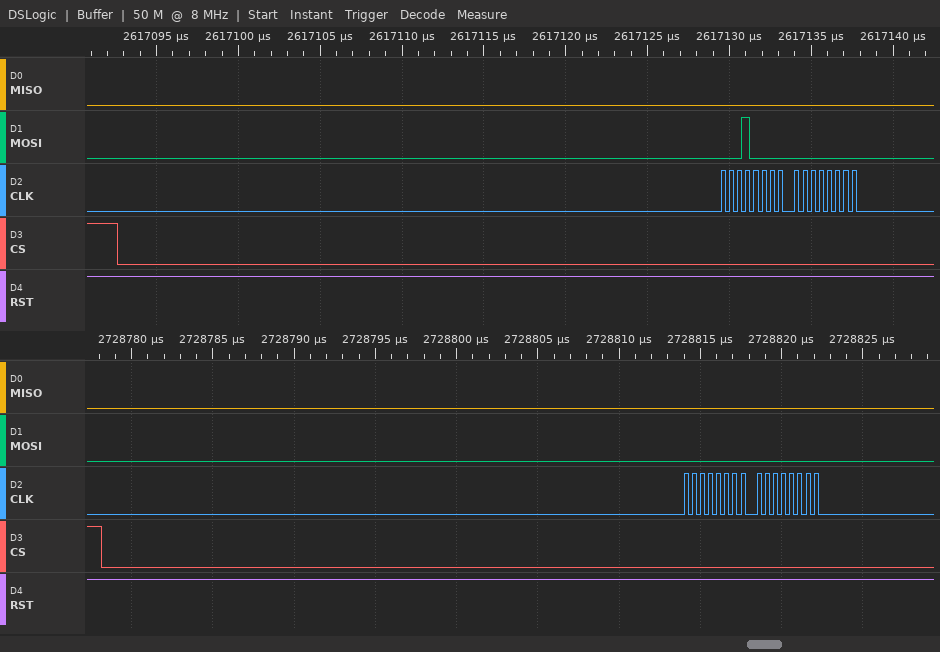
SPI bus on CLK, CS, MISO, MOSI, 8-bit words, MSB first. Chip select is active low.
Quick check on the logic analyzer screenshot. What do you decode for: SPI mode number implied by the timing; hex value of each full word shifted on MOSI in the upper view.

0
10, 00
